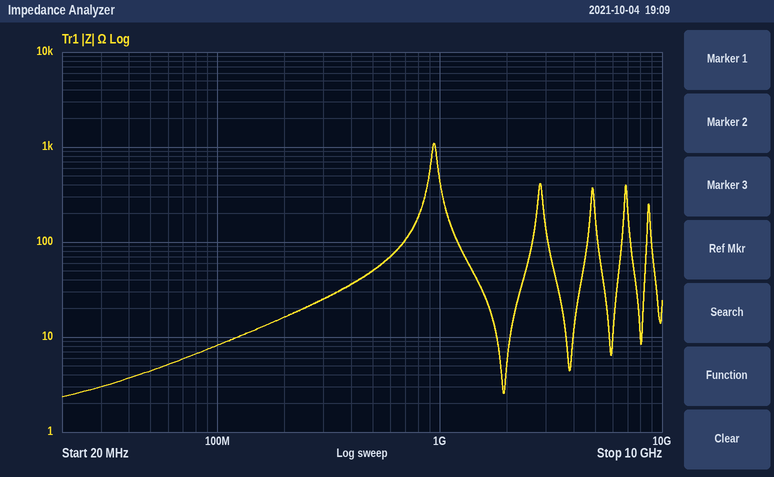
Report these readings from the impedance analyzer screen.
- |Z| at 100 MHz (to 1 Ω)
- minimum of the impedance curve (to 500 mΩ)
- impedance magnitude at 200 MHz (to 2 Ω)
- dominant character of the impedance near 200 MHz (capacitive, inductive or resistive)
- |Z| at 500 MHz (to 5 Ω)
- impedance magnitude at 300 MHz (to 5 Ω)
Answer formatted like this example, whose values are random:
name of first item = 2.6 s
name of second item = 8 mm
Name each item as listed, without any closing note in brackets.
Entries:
|Z| at 100 MHz = 8 Ω
minimum of the impedance curve = 2.5 Ω
impedance magnitude at 200 MHz = 16 Ω
dominant character of the impedance near 200 MHz = inductive
|Z| at 500 MHz = 50 Ω
impedance magnitude at 300 MHz = 25 Ω
